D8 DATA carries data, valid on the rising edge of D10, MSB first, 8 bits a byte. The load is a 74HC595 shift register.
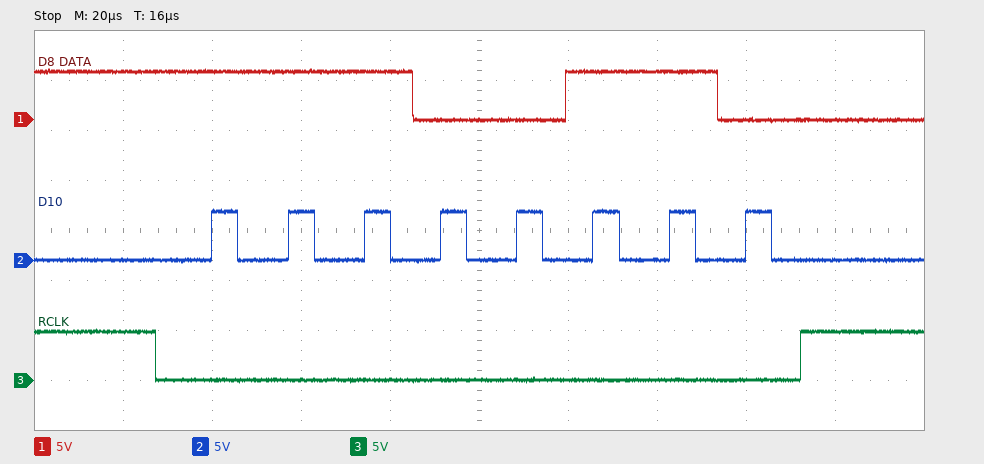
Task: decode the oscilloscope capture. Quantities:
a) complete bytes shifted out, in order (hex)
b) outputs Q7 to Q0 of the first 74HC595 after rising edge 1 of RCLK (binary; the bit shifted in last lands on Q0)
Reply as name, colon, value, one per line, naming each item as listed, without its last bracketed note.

complete bytes shifted out, in order: E6
outputs Q7 to Q0 of the first 74HC595 after rising edge 1 of RCLK: 11100110
